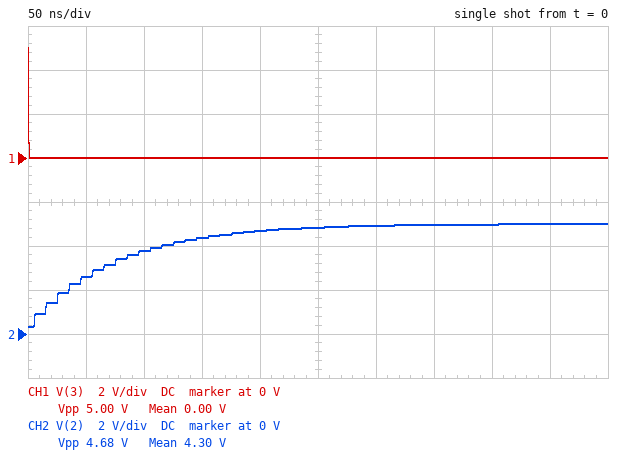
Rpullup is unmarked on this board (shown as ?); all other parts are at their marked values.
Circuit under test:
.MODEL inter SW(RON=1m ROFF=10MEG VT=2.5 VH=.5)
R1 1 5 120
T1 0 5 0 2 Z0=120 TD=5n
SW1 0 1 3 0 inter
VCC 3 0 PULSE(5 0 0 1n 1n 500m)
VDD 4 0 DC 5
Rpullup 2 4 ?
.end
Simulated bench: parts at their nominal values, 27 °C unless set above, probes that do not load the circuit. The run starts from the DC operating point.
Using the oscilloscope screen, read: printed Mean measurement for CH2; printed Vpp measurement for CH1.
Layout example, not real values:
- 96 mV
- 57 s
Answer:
- 4.30 V
- 5.00 V
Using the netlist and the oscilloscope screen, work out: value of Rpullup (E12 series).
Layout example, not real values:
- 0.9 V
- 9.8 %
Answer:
- 1.8 kΩ
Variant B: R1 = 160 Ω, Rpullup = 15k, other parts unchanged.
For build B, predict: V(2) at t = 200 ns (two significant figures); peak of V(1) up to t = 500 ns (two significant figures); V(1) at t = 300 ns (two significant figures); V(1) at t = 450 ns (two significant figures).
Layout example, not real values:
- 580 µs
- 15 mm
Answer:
- 1.4 V
- 2.8 V
- 1.9 V
- 2.6 V
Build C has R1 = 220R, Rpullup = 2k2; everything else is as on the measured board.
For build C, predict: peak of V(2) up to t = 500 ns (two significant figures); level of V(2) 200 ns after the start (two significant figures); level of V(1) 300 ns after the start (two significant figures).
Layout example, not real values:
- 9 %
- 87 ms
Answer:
- 5.0 V
- 4.5 V
- 4.8 V
